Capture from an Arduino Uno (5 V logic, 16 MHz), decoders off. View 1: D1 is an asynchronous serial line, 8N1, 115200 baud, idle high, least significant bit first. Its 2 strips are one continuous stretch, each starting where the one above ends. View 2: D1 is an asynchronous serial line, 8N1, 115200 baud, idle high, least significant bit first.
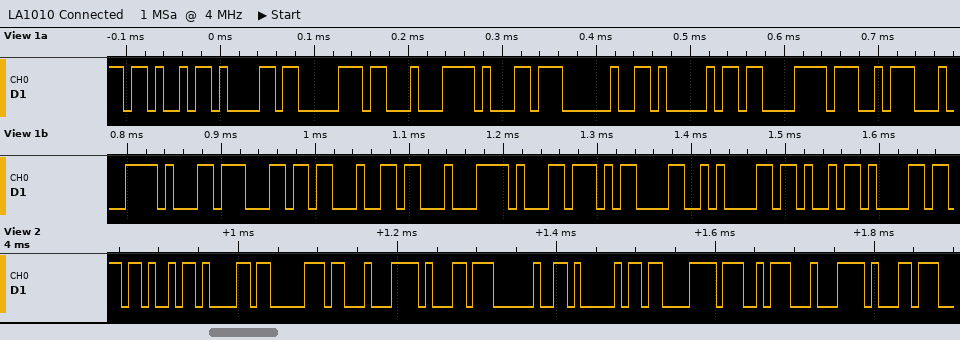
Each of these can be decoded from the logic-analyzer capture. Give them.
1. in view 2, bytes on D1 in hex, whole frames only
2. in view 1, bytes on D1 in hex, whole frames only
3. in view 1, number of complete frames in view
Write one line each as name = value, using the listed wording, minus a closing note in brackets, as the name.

in view 2, bytes on D1 in hex, whole frames only = 4B 61 70 C4 B1 20 41 C3 A7 C4 B1
in view 1, bytes on D1 in hex, whole frames only = 4B 61 70 C4 B1 20 41 C3 A7 C4 B1 6C 64 C4 B1 0D 0A 4B 61
in view 1, number of complete frames in view = 19
